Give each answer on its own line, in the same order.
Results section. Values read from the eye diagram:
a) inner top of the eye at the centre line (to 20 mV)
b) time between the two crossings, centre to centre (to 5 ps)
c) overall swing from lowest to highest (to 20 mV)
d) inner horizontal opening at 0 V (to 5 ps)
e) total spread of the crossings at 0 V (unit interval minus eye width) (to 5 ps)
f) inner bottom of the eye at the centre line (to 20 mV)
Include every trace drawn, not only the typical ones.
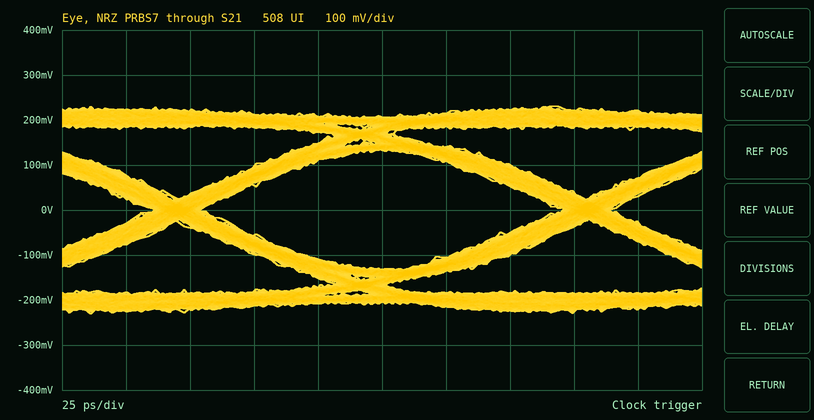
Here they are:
140 mV
160 ps
460 mV
140 ps
20 ps
-140 mV
